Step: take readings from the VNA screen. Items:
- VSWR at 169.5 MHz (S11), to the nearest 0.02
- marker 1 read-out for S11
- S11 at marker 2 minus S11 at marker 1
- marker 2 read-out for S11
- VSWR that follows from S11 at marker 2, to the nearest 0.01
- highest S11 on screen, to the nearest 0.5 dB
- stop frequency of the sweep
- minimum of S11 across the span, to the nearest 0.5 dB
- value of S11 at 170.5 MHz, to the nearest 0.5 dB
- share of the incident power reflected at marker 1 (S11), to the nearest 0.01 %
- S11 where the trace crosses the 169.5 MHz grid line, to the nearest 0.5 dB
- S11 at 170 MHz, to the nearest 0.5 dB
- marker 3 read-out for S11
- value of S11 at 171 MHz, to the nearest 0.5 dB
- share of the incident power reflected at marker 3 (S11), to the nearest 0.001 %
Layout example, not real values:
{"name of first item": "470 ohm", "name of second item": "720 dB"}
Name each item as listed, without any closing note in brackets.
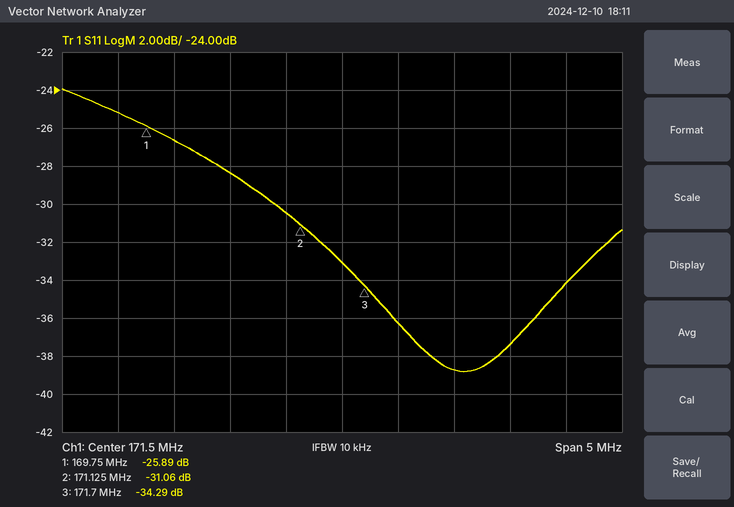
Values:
{"VSWR at 169.5 MHz (S11), to the nearest 0.02": "1.12", "marker 1 read-out for S11": "-25.89 dB", "S11 at marker 2 minus S11 at marker 1": "-5.17 dB", "marker 2 read-out for S11": "-31.06 dB", "VSWR that follows from S11 at marker 2, to the nearest 0.01": "1.06", "highest S11 on screen, to the nearest 0.5 dB": "-24.0 dB", "stop frequency of the sweep": "174 MHz", "minimum of S11 across the span, to the nearest 0.5 dB": "-39.0 dB", "value of S11 at 170.5 MHz, to the nearest 0.5 dB": "-28.5 dB", "share of the incident power reflected at marker 1 (S11), to the nearest 0.01 %": "0.26 %", "S11 where the trace crosses the 169.5 MHz grid line, to the nearest 0.5 dB": "-25.0 dB", "S11 at 170 MHz, to the nearest 0.5 dB": "-26.5 dB", "marker 3 read-out for S11": "-34.29 dB", "value of S11 at 171 MHz, to the nearest 0.5 dB": "-30.5 dB", "share of the incident power reflected at marker 3 (S11), to the nearest 0.001 %": "0.037 %"}
